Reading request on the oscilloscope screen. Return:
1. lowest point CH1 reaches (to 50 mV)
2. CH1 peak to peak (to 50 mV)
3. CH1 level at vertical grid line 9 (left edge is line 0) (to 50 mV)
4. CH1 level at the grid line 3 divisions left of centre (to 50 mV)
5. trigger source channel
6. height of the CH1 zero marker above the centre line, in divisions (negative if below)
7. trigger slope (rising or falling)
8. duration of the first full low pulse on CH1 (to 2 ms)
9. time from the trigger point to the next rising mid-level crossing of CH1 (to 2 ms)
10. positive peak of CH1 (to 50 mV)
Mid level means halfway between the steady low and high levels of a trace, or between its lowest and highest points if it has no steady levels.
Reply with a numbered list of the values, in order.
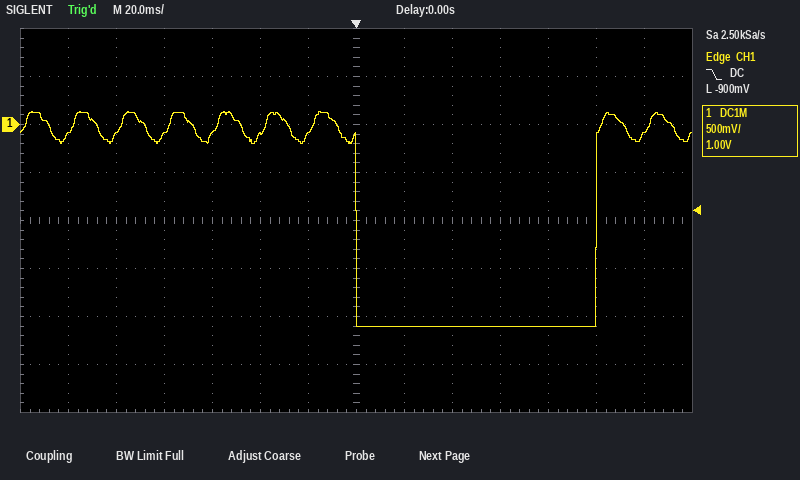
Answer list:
1. -2.10 V
2. 2.25 V
3. -2.10 V
4. -100 mV
5. CH1
6. +2.0 div
7. falling
8. 100 ms
9. 100 ms
10. 150 mV
